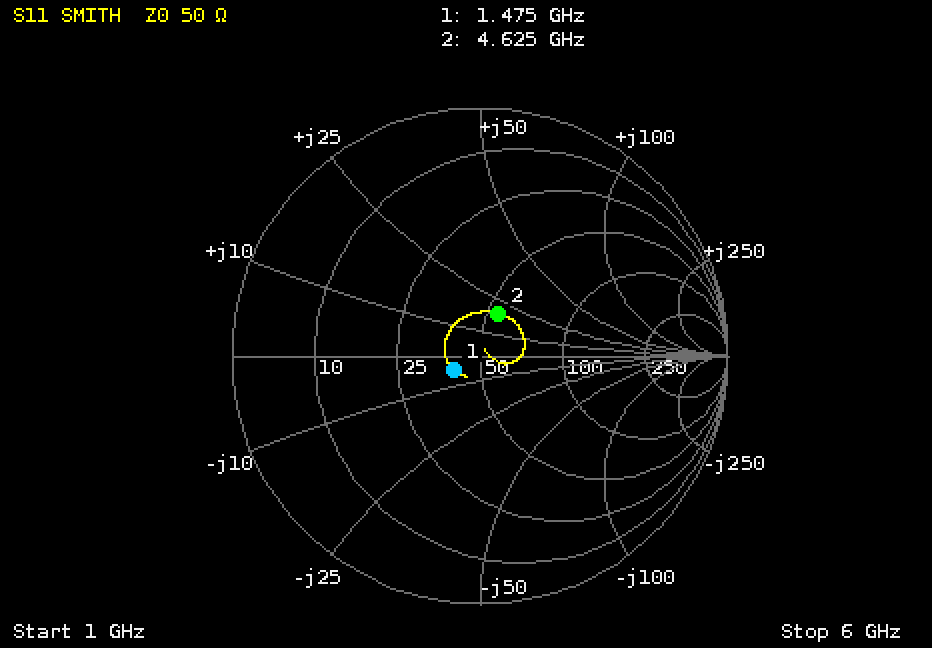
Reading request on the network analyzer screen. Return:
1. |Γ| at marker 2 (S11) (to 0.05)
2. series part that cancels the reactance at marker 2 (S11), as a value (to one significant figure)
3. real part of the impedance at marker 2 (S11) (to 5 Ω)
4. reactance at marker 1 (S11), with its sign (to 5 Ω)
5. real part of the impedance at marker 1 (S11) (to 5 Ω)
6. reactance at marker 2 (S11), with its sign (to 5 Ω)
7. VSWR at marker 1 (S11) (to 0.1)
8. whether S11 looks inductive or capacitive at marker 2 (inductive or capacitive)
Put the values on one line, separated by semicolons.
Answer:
0.20; 2 pF; 55 Ω; -5 Ω; 40 Ω; +20 Ω; 1.3; inductive
